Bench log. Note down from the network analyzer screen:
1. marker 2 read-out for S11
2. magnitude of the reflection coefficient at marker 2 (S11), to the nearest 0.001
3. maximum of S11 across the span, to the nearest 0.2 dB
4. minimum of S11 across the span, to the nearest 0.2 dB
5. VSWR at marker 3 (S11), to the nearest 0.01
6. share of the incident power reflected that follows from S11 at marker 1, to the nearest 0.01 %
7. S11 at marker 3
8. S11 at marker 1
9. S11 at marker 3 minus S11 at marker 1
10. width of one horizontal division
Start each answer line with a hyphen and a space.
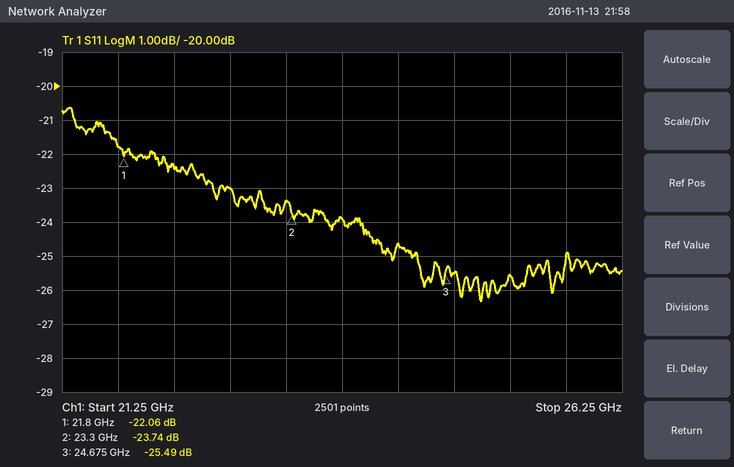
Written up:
- -23.74 dB
- 0.065
- -20.6 dB
- -26.4 dB
- 1.11
- 0.62 %
- -25.49 dB
- -22.06 dB
- -3.43 dB
- 500 MHz
